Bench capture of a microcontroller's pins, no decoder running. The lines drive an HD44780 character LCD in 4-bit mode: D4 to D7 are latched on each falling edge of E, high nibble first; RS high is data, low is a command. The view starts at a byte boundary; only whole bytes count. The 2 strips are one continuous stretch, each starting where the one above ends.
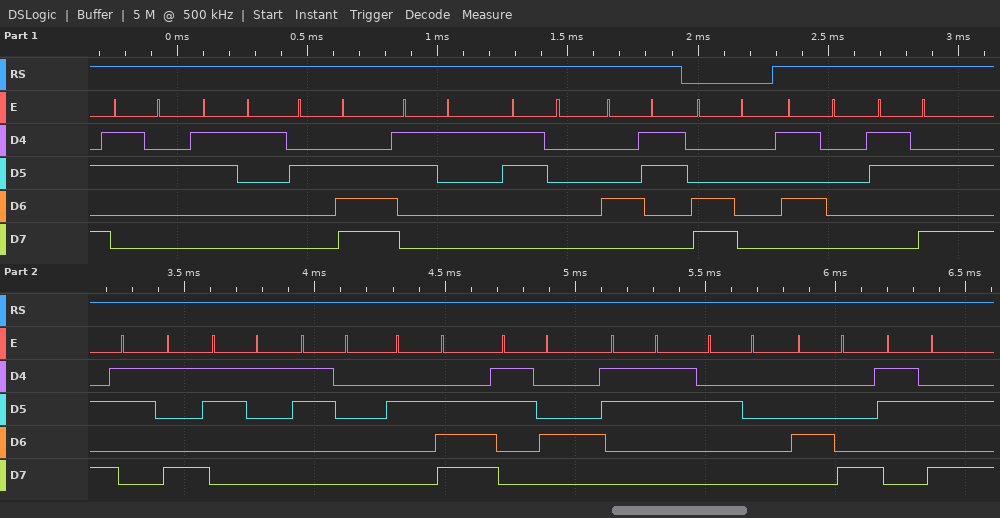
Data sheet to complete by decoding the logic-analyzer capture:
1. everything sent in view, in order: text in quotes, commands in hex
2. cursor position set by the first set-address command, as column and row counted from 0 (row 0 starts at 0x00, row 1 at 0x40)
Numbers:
"21.10C" 0xC0 "P:910.43 H:"
column 0, row 1
